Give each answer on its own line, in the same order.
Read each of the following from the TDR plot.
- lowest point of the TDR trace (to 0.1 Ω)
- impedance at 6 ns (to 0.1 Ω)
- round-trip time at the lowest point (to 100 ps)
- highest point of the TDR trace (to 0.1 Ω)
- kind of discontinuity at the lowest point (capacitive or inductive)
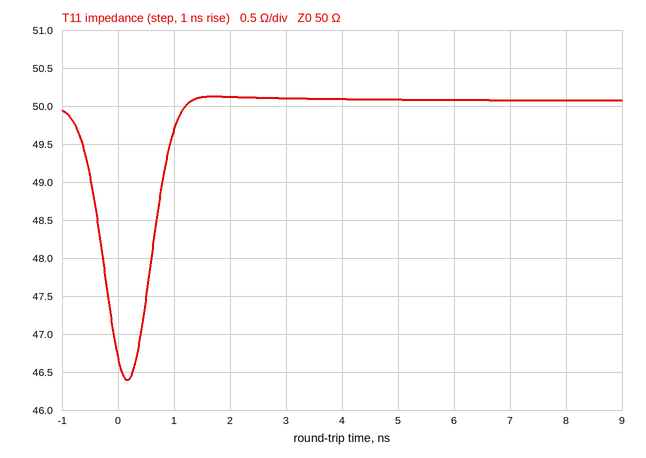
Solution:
46.4 Ω
50.1 Ω
200 ps
50.1 Ω
capacitive
